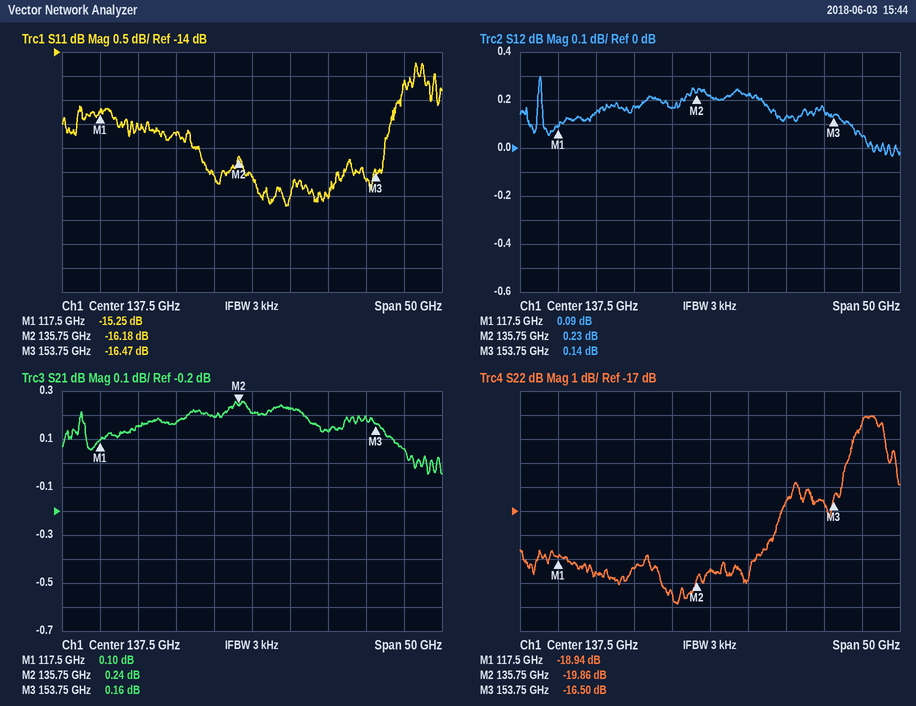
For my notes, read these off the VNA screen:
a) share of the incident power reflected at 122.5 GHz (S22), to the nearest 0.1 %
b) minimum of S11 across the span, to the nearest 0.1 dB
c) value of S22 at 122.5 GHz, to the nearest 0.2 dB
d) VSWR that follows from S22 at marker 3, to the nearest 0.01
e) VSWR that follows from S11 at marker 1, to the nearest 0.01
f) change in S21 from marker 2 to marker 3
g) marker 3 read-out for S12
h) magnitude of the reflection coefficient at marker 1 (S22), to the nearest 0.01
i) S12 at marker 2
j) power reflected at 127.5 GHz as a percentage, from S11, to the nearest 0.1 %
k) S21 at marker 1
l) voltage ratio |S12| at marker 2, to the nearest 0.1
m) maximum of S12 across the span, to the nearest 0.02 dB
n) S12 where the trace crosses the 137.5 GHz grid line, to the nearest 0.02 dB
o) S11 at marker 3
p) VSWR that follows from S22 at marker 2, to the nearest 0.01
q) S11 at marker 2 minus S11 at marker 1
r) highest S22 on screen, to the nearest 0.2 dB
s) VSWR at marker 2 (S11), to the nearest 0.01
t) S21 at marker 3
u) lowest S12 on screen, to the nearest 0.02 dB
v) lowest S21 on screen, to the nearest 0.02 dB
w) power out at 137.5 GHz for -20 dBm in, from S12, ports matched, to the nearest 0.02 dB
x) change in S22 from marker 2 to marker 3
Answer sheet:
1.1 %
-17.2 dB
-19.6 dB
1.35
1.42
-0.08 dB
0.14 dB
0.11
0.23 dB
2.7 %
0.10 dB
1.0
0.30 dB
0.22 dB
-16.47 dB
1.23
-0.93 dB
-13.0 dB
1.37
0.16 dB
-0.04 dB
-0.04 dB
-19.78 dBm
3.36 dB
